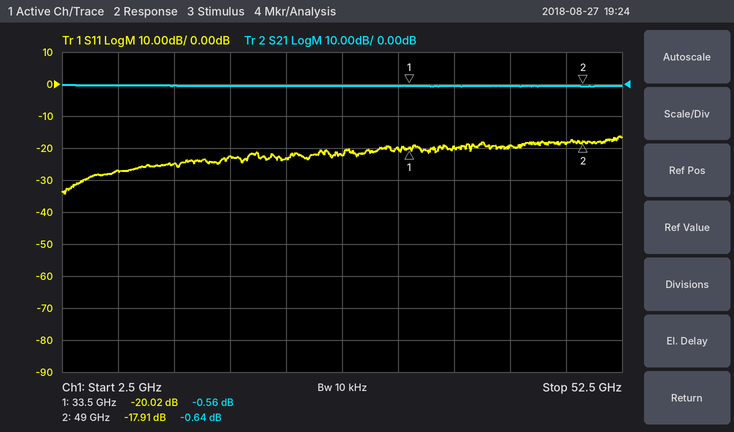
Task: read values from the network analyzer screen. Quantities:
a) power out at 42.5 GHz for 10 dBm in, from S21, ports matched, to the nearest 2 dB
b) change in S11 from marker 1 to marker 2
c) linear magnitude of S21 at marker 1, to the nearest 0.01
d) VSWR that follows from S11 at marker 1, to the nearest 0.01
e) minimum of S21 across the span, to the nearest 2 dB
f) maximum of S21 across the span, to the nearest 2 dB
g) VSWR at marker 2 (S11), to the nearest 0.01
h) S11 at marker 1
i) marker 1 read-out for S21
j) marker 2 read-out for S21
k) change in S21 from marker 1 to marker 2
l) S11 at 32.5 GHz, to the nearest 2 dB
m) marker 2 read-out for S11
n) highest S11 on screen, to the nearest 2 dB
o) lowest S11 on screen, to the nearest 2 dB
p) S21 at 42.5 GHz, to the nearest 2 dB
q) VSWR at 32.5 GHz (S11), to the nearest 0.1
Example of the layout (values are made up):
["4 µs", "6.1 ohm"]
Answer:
["10 dBm", "2.11 dB", "0.94", "1.22", "0 dB", "0 dB", "1.29", "-20.02 dB", "-0.56 dB", "-0.64 dB", "-0.08 dB", "-20 dB", "-17.91 dB", "-16 dB", "-34 dB", "0 dB", "1.2"]
